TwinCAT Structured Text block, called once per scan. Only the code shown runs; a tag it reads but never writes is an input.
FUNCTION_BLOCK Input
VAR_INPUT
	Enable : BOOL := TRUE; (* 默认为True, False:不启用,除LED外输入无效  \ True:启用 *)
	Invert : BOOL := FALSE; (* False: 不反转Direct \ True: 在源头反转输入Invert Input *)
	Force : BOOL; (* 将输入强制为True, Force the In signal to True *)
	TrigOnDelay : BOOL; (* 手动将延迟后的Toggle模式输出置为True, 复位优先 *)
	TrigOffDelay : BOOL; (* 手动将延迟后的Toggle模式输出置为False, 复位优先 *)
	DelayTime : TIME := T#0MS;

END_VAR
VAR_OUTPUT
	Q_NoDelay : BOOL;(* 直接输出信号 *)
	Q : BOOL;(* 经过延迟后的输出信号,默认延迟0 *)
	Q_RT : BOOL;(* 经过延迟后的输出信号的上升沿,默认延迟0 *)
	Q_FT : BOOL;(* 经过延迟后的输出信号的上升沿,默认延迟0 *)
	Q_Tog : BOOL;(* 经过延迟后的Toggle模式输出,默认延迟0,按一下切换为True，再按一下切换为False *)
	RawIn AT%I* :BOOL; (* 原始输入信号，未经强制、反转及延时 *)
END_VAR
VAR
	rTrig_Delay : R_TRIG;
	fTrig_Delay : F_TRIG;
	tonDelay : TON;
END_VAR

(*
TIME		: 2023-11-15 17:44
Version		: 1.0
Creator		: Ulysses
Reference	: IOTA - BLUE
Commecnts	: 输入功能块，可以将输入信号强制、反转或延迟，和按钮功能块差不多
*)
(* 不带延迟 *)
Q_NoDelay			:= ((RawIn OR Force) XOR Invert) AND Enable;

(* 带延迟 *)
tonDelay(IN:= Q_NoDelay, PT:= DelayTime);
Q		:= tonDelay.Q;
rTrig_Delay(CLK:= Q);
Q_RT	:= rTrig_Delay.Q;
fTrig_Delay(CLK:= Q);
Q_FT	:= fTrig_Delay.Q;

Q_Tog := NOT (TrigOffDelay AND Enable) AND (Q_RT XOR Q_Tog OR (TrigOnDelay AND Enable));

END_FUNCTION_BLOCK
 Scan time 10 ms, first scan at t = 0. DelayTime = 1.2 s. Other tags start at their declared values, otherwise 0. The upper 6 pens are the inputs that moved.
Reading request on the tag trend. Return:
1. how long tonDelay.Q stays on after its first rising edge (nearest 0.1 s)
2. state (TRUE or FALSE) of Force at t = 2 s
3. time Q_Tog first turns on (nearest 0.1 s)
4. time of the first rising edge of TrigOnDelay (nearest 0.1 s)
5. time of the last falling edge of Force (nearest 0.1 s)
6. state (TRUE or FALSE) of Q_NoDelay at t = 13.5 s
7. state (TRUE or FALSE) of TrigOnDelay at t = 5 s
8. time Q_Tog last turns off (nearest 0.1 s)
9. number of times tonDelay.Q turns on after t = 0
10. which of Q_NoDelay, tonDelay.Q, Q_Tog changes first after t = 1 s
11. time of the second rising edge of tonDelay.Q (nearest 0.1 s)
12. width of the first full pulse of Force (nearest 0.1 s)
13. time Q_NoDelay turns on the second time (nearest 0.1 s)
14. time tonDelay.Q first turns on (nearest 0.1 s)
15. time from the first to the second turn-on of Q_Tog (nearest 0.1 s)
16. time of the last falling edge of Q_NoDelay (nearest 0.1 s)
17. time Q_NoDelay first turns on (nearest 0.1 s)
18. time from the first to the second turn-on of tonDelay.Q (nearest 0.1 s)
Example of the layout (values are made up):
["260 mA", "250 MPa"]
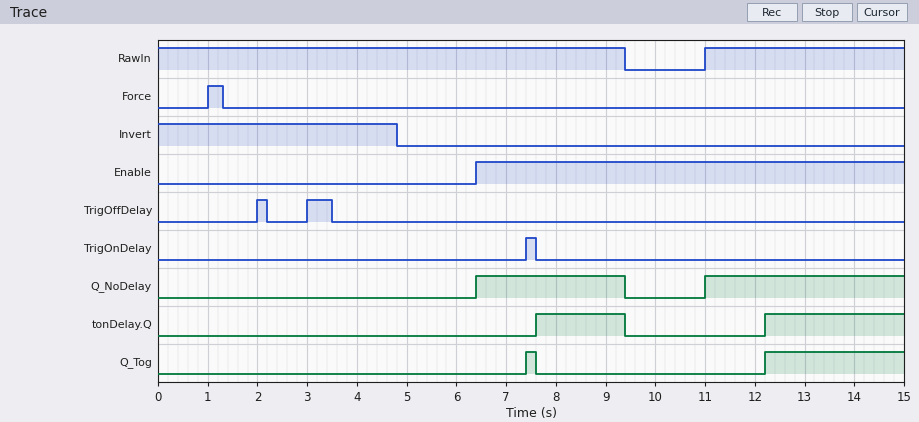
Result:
["1.8 s", "FALSE", "7.4 s", "7.4 s", "1.3 s", "TRUE", "FALSE", "7.6 s", "2", "Q_NoDelay", "12.2 s", "0.3 s", "11.0 s", "7.6 s", "4.8 s", "9.4 s", "6.4 s", "4.6 s"]
